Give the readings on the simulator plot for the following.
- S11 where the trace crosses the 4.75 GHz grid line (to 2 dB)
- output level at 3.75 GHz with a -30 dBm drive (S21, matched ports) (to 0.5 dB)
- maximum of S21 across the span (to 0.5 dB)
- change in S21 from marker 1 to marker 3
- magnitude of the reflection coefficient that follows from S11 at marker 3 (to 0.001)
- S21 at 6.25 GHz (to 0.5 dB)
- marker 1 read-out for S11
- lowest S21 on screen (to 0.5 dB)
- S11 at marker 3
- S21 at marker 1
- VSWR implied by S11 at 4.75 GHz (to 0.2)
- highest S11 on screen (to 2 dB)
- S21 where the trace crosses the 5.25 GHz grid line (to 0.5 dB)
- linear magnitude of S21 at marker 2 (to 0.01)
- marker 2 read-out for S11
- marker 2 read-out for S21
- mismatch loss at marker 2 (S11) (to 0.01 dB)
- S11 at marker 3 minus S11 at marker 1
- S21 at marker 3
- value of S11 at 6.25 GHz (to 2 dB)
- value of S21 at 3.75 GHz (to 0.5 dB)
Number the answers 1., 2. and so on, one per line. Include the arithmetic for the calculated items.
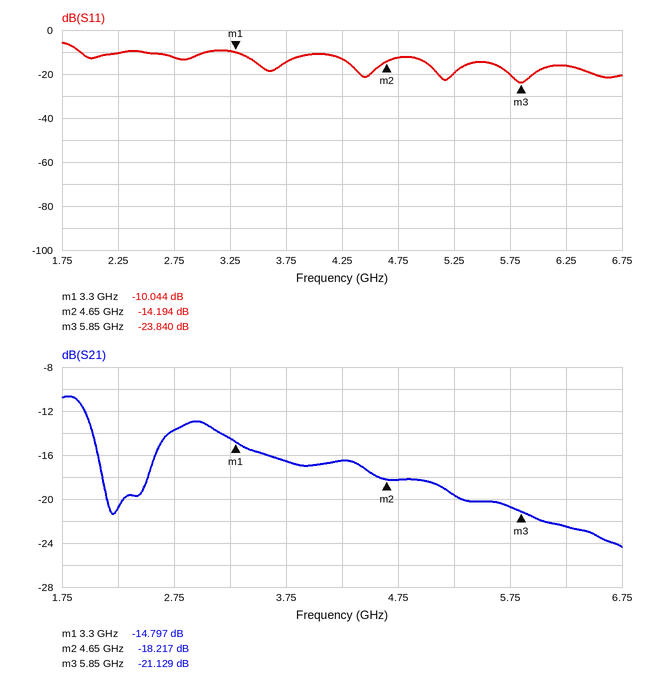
1. -12 dB
2. -30 dBm + (-16.5 dB) = -46.5 dBm
3. -10.5 dB
4. -21.129 − (-14.797) = -6.332 dB
5. 10^(-23.84/20) ≈ 0.064
6. -22.5 dB
7. -10.044 dB
8. -24.5 dB
9. -23.840 dB
10. -14.797 dB
11. |Γ| = 10^(-12/20) = 0.2512; VSWR = (1 + 0.2512)/(1 − 0.2512) ≈ 1.67, so 1.6 to the nearest 0.2
12. -6 dB
13. -19.5 dB
14. 10^(-18.217/20) ≈ 0.12
15. -14.194 dB
16. -18.217 dB
17. −10 log10(1 − 10^(-14.194/10)) ≈ 0.17 dB
18. -23.84 − (-10.044) = -13.796 dB
19. -21.129 dB
20. -16 dB
21. -16.5 dB
